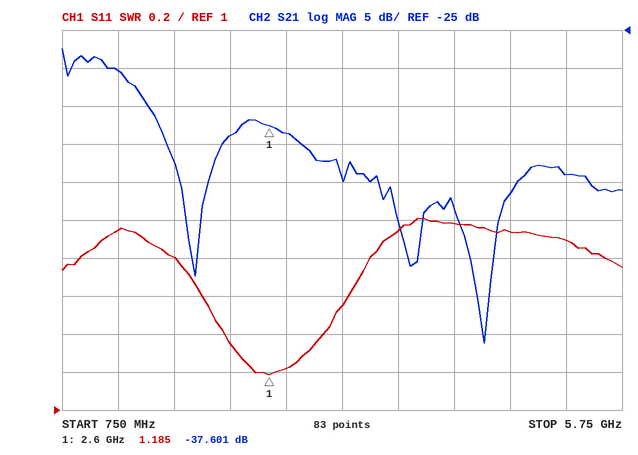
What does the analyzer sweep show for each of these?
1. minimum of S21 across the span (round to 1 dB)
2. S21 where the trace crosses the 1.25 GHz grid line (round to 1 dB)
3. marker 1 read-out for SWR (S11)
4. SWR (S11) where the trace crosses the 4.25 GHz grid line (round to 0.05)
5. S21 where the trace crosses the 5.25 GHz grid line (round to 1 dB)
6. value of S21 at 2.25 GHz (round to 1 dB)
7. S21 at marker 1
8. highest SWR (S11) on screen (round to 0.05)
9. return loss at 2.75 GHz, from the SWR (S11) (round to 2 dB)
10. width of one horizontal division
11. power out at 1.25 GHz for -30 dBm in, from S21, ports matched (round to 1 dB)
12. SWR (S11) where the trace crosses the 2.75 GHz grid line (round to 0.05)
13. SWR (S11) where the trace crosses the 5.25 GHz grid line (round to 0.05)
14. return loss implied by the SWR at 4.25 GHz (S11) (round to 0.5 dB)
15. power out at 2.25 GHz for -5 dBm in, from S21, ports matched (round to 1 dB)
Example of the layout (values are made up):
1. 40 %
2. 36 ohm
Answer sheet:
1. -66 dB
2. -30 dB
3. 1.185
4. 2.00
5. -44 dB
6. -39 dB
7. -37.601 dB
8. 2.00
9. 20 dB
10. 500 MHz
11. -60 dBm
12. 1.20
13. 1.90
14. 9.5 dB
15. -44 dBm
